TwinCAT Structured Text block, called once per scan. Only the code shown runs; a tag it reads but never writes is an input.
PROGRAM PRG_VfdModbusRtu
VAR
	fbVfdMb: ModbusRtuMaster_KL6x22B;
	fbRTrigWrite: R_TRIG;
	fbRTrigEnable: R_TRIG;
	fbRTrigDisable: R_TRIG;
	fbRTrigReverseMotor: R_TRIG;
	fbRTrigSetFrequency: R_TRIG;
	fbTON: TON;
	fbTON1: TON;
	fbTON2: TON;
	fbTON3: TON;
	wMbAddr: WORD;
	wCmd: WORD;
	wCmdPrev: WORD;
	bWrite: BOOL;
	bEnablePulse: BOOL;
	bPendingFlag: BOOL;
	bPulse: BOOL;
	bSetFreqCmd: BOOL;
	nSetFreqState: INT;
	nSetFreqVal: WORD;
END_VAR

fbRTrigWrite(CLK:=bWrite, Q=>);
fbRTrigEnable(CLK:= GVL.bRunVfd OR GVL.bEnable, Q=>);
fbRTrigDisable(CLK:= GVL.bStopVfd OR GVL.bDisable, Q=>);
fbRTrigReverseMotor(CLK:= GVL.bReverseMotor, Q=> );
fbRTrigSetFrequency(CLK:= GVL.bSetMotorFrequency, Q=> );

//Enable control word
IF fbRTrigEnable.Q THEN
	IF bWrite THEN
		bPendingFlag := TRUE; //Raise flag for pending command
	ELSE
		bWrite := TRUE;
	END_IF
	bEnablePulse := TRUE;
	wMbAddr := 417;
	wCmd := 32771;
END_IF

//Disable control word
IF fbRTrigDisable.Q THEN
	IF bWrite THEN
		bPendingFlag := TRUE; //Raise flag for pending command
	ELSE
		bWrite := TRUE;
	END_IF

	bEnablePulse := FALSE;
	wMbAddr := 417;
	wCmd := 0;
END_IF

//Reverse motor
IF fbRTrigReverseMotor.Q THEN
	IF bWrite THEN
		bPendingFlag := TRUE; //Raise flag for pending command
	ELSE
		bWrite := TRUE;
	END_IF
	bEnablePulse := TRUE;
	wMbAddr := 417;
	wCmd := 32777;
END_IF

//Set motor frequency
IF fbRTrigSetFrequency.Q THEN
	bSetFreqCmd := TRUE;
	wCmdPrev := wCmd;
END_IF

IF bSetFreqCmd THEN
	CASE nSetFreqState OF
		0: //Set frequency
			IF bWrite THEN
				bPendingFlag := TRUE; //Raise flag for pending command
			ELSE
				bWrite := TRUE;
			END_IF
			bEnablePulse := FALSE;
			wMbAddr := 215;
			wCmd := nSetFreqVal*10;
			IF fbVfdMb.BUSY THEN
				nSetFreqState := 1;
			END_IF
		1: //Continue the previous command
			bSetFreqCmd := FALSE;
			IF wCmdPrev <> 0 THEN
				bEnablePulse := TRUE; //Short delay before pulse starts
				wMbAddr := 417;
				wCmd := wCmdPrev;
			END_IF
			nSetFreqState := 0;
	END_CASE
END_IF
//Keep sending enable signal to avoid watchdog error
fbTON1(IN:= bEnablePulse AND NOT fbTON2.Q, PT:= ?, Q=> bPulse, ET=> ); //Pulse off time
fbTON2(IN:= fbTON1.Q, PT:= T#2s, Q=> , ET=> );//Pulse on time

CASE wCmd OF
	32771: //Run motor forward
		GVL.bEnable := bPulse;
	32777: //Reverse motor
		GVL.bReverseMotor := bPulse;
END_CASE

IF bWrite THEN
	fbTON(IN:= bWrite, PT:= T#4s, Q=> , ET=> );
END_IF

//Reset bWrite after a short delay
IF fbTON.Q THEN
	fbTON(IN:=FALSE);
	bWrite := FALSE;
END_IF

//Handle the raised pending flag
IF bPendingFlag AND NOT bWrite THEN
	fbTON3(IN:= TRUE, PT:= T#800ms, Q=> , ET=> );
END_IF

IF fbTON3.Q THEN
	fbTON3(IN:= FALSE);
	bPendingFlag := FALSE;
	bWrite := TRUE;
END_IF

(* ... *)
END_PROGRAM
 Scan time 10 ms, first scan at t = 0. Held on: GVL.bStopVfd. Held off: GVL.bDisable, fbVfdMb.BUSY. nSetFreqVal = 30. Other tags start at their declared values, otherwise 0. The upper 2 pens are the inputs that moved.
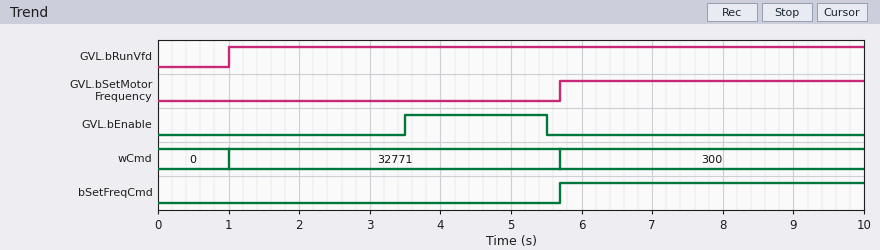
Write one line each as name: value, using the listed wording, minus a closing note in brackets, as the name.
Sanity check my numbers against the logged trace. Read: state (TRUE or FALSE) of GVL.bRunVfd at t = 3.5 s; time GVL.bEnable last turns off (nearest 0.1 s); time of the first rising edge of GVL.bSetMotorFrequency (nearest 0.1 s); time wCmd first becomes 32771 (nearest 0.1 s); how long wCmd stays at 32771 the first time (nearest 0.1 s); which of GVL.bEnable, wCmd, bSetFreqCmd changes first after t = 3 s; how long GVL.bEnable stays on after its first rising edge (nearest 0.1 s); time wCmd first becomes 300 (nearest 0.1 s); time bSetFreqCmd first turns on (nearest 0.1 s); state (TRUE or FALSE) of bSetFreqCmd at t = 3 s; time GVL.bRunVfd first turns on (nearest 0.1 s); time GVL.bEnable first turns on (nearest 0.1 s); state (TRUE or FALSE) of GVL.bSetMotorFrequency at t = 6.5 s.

state (TRUE or FALSE) of GVL.bRunVfd at t = 3.5 s: TRUE
time GVL.bEnable last turns off: 5.5 s
time of the first rising edge of GVL.bSetMotorFrequency: 5.7 s
time wCmd first becomes 32771: 1.0 s
how long wCmd stays at 32771 the first time: 4.7 s
which of GVL.bEnable, wCmd, bSetFreqCmd changes first after t = 3 s: GVL.bEnable
how long GVL.bEnable stays on after its first rising edge: 2.0 s
time wCmd first becomes 300: 5.7 s
time bSetFreqCmd first turns on: 5.7 s
state (TRUE or FALSE) of bSetFreqCmd at t = 3 s: FALSE
time GVL.bRunVfd first turns on: 1.0 s
time GVL.bEnable first turns on: 3.5 s
state (TRUE or FALSE) of GVL.bSetMotorFrequency at t = 6.5 s: TRUE
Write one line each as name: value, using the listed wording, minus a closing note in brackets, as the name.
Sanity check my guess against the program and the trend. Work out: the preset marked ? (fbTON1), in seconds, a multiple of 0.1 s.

the preset marked ? (fbTON1), in seconds, a multiple of 0.1 s: 2.5 s
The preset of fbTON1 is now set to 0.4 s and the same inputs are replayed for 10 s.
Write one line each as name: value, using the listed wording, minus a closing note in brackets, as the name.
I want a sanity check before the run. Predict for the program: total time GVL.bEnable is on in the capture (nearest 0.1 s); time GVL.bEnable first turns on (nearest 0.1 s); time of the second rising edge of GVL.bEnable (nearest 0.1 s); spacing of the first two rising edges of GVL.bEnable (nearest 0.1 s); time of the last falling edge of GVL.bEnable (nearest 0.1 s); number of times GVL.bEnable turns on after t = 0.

total time GVL.bEnable is on in the capture: 8.2 s
time GVL.bEnable first turns on: 1.4 s
time of the second rising edge of GVL.bEnable: 3.8 s
spacing of the first two rising edges of GVL.bEnable: 2.4 s
time of the last falling edge of GVL.bEnable: 3.4 s
number of times GVL.bEnable turns on after t = 0: 2
